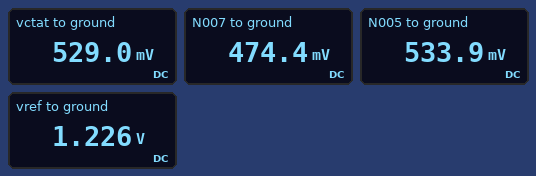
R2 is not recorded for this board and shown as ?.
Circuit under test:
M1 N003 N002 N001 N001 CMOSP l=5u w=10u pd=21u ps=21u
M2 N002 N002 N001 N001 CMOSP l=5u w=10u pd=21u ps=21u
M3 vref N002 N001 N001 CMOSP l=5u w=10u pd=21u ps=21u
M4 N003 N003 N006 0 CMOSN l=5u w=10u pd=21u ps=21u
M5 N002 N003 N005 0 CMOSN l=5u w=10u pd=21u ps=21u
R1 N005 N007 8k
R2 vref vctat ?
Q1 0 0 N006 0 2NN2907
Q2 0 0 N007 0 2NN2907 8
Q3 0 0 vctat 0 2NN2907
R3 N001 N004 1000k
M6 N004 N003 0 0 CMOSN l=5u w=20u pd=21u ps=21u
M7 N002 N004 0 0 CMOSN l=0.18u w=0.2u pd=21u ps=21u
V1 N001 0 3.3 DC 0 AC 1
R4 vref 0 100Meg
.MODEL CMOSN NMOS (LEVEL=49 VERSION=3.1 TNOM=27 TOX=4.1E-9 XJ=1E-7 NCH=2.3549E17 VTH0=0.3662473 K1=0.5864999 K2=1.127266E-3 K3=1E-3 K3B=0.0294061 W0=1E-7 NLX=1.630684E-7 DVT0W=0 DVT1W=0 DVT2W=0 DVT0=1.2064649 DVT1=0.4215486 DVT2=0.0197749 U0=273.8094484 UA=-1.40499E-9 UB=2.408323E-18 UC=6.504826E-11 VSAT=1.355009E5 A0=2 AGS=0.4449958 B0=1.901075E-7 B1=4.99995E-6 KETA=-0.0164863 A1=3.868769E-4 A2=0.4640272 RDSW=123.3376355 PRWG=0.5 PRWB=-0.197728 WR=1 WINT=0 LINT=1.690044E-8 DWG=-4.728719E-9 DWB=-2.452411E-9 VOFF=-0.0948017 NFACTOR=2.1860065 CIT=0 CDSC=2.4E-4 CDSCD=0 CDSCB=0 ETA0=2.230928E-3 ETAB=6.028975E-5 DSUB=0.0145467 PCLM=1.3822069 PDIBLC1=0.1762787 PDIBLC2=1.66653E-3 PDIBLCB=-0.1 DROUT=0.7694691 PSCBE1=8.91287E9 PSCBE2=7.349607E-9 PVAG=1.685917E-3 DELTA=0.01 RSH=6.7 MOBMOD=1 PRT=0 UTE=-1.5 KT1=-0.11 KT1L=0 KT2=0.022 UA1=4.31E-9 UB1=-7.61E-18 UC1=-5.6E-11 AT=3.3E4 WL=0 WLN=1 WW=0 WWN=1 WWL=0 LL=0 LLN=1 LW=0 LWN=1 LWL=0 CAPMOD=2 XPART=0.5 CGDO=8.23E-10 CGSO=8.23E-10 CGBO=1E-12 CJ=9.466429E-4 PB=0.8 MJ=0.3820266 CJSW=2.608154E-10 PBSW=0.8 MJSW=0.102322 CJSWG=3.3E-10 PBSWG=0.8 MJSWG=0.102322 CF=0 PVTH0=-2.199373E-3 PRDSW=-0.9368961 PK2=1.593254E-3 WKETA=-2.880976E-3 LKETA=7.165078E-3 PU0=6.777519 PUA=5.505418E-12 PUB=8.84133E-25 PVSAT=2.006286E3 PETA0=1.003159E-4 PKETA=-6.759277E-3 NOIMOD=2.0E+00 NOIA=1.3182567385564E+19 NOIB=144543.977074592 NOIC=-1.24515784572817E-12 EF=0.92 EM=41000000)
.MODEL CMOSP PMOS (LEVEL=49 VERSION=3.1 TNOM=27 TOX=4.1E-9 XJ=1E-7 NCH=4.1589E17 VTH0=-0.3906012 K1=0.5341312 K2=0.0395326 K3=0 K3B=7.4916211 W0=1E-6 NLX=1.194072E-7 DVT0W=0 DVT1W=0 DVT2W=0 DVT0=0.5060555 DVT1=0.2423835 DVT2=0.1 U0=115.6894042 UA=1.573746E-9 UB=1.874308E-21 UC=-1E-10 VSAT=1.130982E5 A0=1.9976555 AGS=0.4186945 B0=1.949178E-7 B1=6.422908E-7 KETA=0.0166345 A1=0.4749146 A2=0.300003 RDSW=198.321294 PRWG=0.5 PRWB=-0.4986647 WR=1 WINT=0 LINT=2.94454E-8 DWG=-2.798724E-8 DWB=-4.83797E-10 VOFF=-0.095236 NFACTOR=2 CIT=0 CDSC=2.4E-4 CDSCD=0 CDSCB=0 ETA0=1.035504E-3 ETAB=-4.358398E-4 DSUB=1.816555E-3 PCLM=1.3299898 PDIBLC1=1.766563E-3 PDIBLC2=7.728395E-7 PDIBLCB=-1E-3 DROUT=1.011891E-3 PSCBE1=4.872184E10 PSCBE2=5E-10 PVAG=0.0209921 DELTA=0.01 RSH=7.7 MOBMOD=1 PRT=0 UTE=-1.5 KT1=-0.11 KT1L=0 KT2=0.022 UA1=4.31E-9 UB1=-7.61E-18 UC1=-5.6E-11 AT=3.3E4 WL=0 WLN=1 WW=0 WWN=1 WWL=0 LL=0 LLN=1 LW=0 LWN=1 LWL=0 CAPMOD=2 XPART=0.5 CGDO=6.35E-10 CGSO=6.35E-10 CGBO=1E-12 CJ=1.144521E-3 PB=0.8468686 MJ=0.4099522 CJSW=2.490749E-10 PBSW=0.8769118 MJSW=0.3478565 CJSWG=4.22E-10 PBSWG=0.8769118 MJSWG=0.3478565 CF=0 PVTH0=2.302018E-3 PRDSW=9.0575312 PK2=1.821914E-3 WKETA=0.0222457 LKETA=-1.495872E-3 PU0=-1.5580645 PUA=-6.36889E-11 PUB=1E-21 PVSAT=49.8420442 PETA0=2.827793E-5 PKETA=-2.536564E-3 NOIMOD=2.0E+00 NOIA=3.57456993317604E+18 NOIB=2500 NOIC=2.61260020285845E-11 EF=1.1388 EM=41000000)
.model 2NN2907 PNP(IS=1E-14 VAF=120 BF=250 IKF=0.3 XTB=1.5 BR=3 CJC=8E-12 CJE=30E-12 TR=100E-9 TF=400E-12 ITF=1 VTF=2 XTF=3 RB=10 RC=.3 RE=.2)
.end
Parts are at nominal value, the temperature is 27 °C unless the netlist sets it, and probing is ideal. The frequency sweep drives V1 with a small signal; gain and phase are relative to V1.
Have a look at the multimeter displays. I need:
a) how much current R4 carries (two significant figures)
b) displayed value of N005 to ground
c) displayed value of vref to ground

12 nA
533.9 mV
1.226 V
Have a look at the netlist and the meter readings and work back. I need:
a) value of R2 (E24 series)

91 kΩ
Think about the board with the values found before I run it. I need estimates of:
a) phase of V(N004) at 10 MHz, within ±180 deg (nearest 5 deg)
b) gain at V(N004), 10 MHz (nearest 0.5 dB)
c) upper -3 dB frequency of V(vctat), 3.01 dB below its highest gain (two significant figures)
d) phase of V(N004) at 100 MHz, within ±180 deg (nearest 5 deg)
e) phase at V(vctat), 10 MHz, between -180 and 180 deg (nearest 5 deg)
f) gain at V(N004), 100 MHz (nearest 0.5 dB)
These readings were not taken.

20 deg
-59.0 dB
910 kHz
65 deg
-60 deg
-49.5 dB
